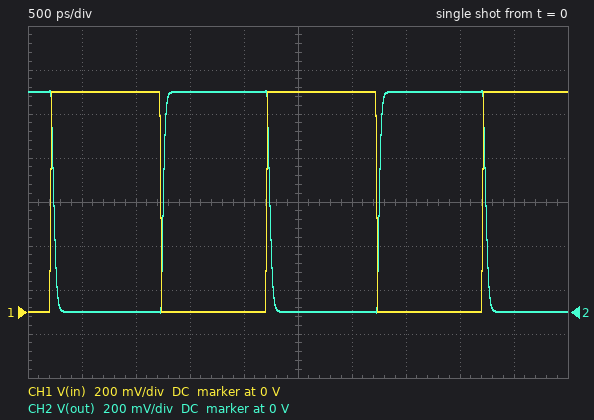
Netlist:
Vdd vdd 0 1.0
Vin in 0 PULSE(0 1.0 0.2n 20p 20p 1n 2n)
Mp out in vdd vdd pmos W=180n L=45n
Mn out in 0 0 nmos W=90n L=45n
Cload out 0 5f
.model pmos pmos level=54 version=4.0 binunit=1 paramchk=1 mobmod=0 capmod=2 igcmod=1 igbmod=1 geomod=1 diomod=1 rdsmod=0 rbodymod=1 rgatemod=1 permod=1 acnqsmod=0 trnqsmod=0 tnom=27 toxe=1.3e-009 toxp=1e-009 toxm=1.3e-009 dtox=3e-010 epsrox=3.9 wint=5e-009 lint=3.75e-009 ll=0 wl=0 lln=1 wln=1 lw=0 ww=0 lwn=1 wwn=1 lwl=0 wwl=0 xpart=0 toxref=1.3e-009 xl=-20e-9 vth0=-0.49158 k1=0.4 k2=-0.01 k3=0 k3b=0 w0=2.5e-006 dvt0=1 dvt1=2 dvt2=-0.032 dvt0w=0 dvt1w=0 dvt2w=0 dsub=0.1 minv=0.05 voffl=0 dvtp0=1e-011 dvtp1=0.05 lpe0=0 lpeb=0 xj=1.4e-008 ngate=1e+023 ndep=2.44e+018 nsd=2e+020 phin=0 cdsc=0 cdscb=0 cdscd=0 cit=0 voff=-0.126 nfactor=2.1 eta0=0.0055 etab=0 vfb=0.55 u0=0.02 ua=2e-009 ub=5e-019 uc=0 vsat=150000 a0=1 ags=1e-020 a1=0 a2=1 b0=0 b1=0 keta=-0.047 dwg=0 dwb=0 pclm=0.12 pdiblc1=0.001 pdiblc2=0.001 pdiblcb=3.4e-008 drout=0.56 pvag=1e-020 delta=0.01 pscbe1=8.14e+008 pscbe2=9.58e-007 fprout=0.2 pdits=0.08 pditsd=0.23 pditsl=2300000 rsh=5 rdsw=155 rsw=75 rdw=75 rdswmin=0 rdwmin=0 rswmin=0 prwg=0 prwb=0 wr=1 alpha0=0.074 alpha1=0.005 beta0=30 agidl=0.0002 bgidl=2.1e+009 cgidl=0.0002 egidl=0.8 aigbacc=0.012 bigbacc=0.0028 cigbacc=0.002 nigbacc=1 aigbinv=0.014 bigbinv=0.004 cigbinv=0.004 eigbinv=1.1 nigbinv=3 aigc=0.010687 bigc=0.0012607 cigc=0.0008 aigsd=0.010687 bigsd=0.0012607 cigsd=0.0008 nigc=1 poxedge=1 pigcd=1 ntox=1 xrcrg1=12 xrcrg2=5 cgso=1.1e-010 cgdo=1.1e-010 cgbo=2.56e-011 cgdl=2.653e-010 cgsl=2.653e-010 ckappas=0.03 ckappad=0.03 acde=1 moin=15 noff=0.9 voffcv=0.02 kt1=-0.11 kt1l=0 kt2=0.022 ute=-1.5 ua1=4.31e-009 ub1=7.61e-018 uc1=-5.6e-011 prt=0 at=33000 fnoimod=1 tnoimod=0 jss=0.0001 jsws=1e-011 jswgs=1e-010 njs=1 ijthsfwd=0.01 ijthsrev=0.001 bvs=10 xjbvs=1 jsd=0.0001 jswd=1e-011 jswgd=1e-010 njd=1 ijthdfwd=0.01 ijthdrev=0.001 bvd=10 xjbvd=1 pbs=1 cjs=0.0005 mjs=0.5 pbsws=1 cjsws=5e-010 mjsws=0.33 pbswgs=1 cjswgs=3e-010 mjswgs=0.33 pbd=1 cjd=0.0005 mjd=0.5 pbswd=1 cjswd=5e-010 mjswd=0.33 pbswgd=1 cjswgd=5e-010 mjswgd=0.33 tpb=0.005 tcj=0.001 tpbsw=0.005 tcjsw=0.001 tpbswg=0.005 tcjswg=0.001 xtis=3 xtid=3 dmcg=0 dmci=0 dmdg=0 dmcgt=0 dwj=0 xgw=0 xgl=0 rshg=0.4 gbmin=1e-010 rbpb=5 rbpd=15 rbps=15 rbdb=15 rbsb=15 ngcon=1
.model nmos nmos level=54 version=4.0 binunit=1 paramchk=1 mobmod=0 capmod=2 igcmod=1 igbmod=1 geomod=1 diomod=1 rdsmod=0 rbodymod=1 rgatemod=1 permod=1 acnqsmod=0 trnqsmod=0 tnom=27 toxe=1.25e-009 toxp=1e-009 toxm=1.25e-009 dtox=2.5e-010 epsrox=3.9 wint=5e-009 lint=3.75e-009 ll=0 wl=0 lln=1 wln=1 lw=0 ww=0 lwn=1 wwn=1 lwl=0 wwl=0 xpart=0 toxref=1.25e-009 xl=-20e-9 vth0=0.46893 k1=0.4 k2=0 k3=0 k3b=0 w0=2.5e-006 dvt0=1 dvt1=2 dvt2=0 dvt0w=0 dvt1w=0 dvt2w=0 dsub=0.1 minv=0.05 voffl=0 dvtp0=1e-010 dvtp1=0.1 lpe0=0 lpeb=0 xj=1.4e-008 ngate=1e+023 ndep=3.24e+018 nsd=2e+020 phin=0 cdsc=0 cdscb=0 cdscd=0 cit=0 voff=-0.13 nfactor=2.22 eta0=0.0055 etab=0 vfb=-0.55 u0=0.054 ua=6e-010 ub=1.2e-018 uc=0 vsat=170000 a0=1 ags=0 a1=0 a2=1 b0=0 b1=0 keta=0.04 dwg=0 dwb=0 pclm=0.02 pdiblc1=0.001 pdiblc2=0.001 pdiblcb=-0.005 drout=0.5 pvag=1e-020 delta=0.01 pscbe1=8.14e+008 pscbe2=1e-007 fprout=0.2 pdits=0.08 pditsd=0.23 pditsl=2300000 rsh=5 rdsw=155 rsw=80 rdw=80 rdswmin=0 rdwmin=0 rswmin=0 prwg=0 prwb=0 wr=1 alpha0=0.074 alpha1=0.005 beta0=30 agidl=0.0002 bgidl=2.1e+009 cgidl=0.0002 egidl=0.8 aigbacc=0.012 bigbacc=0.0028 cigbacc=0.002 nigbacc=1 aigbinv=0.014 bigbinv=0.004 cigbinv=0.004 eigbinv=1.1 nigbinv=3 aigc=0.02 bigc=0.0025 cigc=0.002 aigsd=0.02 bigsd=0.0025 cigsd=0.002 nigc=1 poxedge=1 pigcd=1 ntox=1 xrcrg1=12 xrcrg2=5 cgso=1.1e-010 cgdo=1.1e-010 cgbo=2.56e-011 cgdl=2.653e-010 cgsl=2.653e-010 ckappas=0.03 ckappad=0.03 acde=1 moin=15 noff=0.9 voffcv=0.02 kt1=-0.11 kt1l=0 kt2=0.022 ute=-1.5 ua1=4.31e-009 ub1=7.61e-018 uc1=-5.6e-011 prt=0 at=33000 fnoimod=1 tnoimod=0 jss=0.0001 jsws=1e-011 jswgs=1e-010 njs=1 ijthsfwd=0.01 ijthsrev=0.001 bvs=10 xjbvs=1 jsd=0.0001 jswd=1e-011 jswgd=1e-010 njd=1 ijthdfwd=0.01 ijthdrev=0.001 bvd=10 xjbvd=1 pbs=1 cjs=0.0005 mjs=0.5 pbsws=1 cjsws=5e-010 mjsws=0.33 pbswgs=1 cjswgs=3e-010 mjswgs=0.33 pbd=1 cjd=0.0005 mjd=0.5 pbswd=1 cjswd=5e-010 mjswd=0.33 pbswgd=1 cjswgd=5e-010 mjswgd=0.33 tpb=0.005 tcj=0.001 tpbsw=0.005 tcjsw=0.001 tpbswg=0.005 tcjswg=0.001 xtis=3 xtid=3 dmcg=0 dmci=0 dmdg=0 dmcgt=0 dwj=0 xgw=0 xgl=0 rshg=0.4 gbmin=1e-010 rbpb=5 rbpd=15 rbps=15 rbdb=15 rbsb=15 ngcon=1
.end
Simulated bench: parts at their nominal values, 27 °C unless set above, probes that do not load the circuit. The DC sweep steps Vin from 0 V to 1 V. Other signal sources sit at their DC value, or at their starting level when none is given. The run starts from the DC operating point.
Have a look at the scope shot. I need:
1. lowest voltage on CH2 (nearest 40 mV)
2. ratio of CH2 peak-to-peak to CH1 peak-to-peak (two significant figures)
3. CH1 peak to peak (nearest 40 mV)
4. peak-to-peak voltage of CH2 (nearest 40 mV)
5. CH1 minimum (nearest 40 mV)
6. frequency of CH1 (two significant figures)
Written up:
0 V
1.0
1.00 V
1.00 V
0 V
500 MHz
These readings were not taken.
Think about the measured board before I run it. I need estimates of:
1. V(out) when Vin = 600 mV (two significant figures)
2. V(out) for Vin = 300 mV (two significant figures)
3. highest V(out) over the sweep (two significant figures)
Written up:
43 mV
990 mV
1.0 V
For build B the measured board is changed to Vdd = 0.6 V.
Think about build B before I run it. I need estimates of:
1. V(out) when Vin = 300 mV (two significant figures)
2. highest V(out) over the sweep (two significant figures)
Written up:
160 mV
600 mV
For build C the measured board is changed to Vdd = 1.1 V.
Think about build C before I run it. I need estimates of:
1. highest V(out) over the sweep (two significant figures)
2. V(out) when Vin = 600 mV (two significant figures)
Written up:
1.1 V
240 mV
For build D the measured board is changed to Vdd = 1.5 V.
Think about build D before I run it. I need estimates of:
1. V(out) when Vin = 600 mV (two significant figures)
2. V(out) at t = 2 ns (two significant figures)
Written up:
1.3 V
1.5 V
